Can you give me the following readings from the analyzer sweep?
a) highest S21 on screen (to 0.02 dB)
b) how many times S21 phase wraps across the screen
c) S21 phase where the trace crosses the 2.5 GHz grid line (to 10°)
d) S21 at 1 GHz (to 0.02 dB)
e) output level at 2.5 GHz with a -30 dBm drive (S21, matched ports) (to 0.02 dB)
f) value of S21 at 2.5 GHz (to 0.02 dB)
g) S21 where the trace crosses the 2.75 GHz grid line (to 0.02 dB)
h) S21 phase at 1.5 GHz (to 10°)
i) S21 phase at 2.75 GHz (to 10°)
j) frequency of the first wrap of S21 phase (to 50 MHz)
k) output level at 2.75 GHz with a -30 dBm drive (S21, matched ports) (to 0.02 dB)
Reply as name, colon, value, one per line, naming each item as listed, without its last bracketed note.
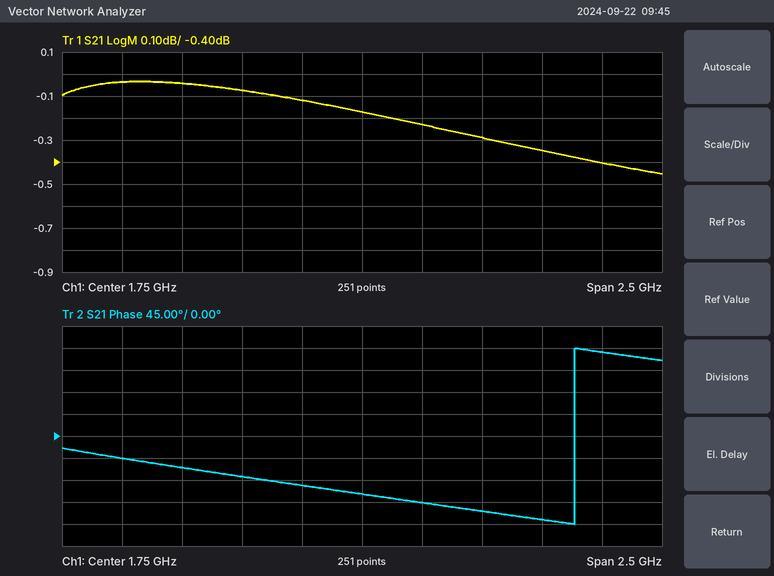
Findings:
highest S21 on screen: -0.04 dB
how many times S21 phase wraps across the screen: 1
S21 phase where the trace crosses the 2.5 GHz grid line: -170°
S21 at 1 GHz: -0.04 dB
output level at 2.5 GHz with a -30 dBm drive (S21, matched ports): -30.34 dBm
value of S21 at 2.5 GHz: -0.34 dB
S21 where the trace crosses the 2.75 GHz grid line: -0.40 dB
S21 phase at 1.5 GHz: -100°
S21 phase at 2.75 GHz: 170°
frequency of the first wrap of S21 phase: 2.65 GHz
output level at 2.75 GHz with a -30 dBm drive (S21, matched ports): -30.40 dBm
